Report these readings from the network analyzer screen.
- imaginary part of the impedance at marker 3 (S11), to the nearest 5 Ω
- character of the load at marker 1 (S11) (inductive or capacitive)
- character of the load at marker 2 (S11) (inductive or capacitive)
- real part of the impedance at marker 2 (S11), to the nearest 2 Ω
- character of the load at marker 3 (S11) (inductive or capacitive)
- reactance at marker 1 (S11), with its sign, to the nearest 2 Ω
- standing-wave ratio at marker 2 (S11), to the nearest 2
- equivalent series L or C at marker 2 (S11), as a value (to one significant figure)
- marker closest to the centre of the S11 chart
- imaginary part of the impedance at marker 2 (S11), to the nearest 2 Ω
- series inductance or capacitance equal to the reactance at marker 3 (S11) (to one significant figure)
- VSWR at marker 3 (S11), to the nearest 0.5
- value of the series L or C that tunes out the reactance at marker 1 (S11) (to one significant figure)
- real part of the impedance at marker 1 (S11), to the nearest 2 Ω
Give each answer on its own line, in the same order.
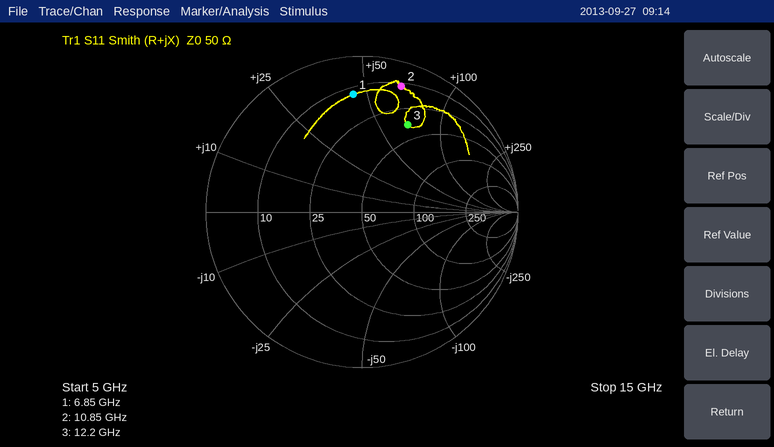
+70 Ω
inductive
inductive
12 Ω
inductive
+44 Ω
12
1.0 nH
marker 3
+66 Ω
900 pH
4.5
500 fF
12 Ω
